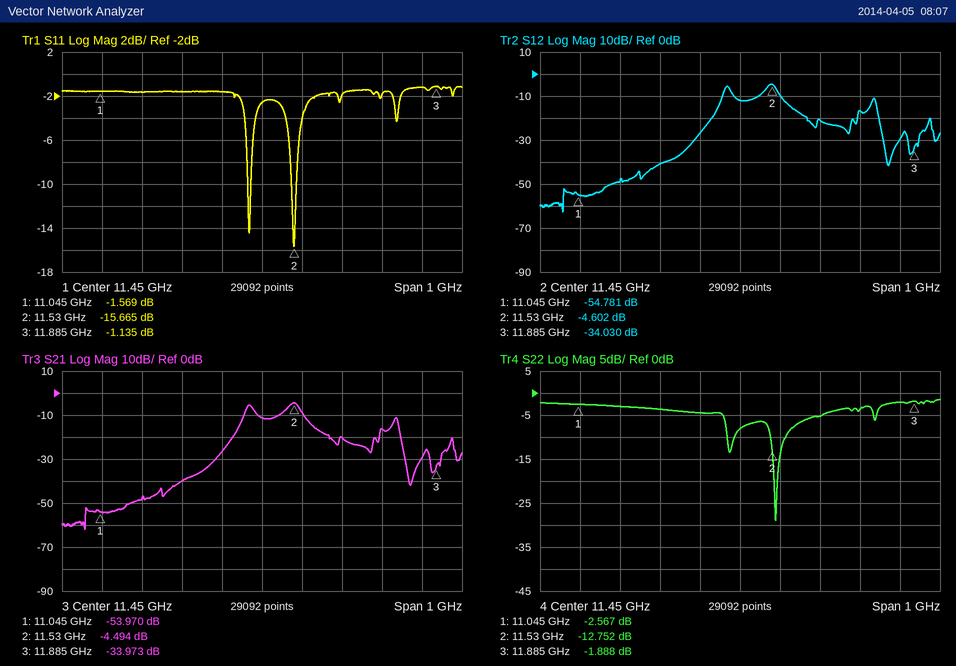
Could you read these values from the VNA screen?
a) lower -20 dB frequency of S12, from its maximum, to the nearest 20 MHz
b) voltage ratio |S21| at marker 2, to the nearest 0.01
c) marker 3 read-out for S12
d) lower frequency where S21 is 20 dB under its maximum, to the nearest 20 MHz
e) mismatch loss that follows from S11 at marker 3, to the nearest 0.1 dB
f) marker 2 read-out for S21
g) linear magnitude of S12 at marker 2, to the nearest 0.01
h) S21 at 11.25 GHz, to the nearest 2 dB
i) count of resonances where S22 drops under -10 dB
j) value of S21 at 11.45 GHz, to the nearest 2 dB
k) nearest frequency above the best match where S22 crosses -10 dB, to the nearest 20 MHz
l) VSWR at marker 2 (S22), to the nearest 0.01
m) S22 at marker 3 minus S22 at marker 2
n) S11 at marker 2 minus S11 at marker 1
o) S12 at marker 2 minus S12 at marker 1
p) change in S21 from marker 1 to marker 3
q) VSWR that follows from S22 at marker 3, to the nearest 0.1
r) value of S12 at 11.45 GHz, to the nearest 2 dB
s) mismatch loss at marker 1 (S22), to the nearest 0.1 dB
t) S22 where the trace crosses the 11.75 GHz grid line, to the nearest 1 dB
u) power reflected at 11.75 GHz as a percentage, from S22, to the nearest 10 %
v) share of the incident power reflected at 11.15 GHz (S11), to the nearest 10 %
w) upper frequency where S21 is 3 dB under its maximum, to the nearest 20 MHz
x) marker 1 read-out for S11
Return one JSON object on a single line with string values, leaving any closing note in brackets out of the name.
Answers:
{"lower -20 dB frequency of S12, from its maximum, to the nearest 20 MHz": "11.36 GHz", "voltage ratio |S21| at marker 2, to the nearest 0.01": "0.60", "marker 3 read-out for S12": "-34.030 dB", "lower frequency where S21 is 20 dB under its maximum, to the nearest 20 MHz": "11.36 GHz", "mismatch loss that follows from S11 at marker 3, to the nearest 0.1 dB": "6.4 dB", "marker 2 read-out for S21": "-4.494 dB", "linear magnitude of S12 at marker 2, to the nearest 0.01": "0.59", "S21 at 11.25 GHz, to the nearest 2 dB": "-40 dB", "count of resonances where S22 drops under -10 dB": "2", "value of S21 at 11.45 GHz, to the nearest 2 dB": "-12 dB", "nearest frequency above the best match where S22 crosses -10 dB, to the nearest 20 MHz": "11.56 GHz", "VSWR at marker 2 (S22), to the nearest 0.01": "1.60", "S22 at marker 3 minus S22 at marker 2": "10.864 dB", "S11 at marker 2 minus S11 at marker 1": "-14.096 dB", "S12 at marker 2 minus S12 at marker 1": "50.179 dB", "change in S21 from marker 1 to marker 3": "19.997 dB", "VSWR that follows from S22 at marker 3, to the nearest 0.1": "9.2", "value of S12 at 11.45 GHz, to the nearest 2 dB": "-12 dB", "mismatch loss at marker 1 (S22), to the nearest 0.1 dB": "3.5 dB", "S22 where the trace crosses the 11.75 GHz grid line, to the nearest 1 dB": "-4 dB", "power reflected at 11.75 GHz as a percentage, from S22, to the nearest 10 %": "40 %", "share of the incident power reflected at 11.15 GHz (S11), to the nearest 10 %": "70 %", "upper frequency where S21 is 3 dB under its maximum, to the nearest 20 MHz": "11.54 GHz", "marker 1 read-out for S11": "-1.569 dB"}
